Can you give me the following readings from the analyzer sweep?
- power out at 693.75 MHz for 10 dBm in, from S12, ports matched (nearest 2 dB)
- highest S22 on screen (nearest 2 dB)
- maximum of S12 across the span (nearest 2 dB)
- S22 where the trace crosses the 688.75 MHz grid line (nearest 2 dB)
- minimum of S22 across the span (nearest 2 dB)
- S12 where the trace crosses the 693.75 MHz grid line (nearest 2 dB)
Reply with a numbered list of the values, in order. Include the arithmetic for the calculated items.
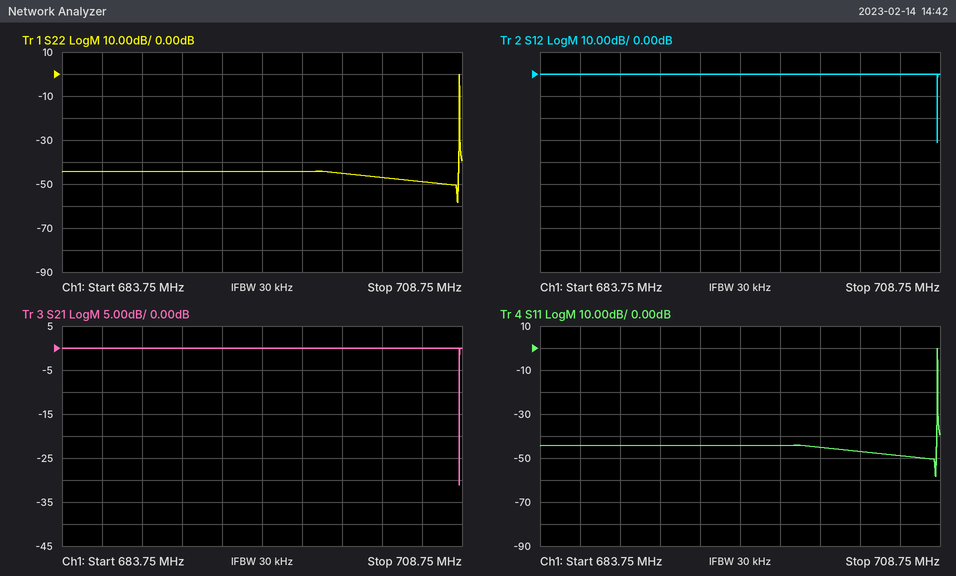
1. 10 dBm + (0 dB) = 10 dBm
2. 0 dB
3. 0 dB
4. -44 dB
5. -58 dB
6. 0 dB
